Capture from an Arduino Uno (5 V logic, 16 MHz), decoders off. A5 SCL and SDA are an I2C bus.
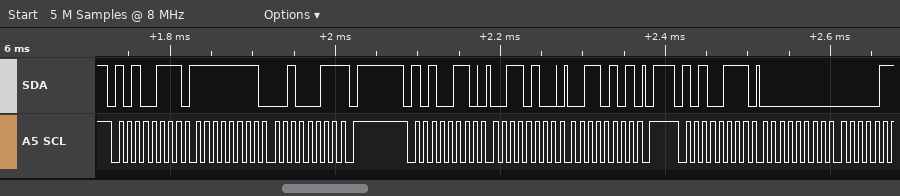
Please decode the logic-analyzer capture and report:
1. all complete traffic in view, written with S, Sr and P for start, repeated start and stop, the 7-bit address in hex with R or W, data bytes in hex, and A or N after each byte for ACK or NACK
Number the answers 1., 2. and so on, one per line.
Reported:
1. S 53R A FF A 23 N P S 53W A 34 A 35 A P S 53R A 00 A
